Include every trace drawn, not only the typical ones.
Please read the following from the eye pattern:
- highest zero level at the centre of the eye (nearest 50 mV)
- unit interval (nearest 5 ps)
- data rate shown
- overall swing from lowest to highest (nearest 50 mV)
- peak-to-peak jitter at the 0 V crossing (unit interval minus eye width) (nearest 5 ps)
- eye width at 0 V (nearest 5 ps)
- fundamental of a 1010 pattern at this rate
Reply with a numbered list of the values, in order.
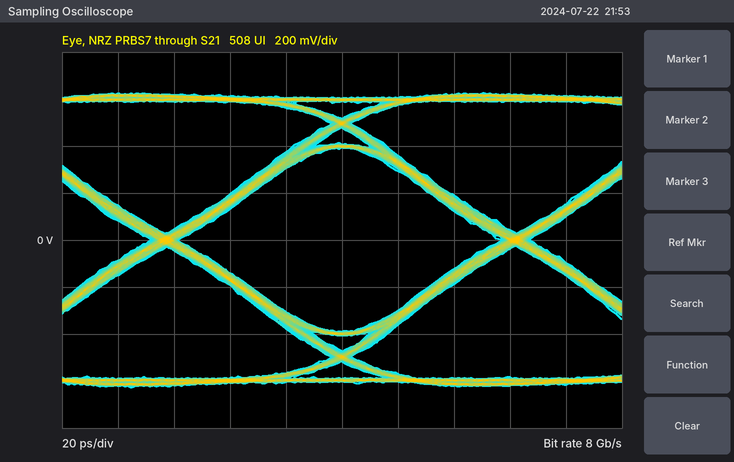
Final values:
1. -400 mV
2. 125 ps
3. 8 Gb/s
4. 1.25 V
5. 10 ps
6. 115 ps
7. 4 GHz
